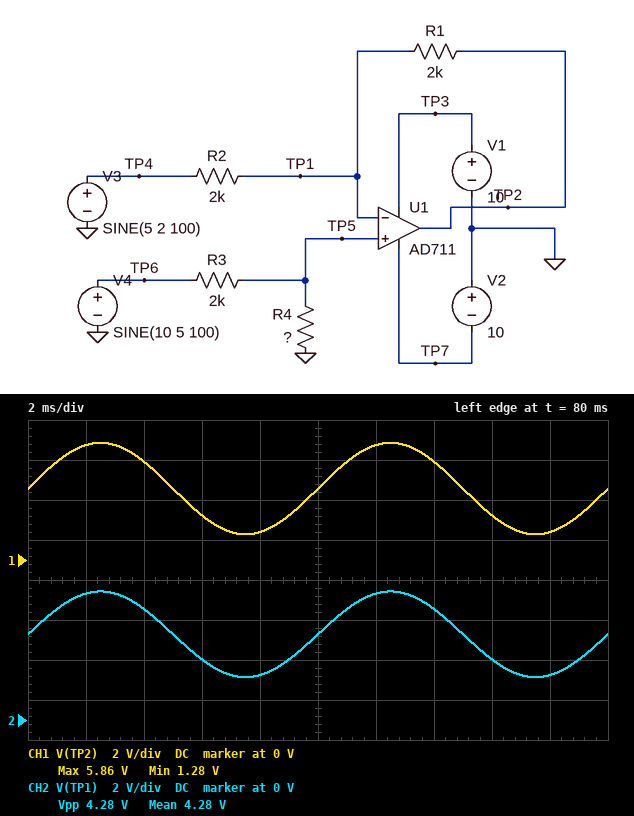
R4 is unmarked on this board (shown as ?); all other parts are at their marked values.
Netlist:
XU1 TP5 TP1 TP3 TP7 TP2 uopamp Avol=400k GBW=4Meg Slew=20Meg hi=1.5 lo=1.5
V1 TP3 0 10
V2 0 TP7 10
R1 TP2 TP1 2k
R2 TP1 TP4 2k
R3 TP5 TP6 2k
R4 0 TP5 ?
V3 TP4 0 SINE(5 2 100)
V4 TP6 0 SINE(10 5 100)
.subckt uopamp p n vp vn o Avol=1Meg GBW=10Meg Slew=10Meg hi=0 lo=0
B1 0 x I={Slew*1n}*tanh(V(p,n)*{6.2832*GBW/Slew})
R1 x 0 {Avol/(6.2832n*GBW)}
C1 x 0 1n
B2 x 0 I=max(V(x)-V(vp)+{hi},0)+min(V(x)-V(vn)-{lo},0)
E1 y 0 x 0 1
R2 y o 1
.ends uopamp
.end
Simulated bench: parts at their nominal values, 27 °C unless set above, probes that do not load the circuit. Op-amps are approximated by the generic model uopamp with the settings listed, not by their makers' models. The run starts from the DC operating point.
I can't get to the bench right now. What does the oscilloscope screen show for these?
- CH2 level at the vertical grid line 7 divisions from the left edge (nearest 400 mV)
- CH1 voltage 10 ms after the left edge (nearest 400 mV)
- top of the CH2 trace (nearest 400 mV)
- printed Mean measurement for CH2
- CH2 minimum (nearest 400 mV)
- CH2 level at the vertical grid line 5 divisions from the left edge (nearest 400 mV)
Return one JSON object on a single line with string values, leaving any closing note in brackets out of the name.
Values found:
{"CH2 level at the vertical grid line 7 divisions from the left edge": "5.6 V", "CH1 voltage 10 ms after the left edge": "3.6 V", "top of the CH2 trace": "6.4 V", "printed Mean measurement for CH2": "4.28 V", "CH2 minimum": "2.0 V", "CH2 level at the vertical grid line 5 divisions from the left edge": "4.4 V"}
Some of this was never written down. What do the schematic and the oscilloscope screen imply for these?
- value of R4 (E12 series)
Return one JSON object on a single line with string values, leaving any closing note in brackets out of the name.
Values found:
{"value of R4": "1.5 kΩ"}
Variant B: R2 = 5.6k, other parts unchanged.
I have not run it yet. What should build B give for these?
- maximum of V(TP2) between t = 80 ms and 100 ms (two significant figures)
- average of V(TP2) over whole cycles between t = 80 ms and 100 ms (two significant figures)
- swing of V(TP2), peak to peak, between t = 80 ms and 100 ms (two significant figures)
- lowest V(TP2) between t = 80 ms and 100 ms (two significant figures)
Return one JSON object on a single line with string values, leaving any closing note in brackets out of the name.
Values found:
{"maximum of V(TP2) between t = 80 ms and 100 ms": "6.2 V", "average of V(TP2) over whole cycles between t = 80 ms and 100 ms": "4.0 V", "swing of V(TP2), peak to peak, between t = 80 ms and 100 ms": "4.4 V", "lowest V(TP2) between t = 80 ms and 100 ms": "1.8 V"}
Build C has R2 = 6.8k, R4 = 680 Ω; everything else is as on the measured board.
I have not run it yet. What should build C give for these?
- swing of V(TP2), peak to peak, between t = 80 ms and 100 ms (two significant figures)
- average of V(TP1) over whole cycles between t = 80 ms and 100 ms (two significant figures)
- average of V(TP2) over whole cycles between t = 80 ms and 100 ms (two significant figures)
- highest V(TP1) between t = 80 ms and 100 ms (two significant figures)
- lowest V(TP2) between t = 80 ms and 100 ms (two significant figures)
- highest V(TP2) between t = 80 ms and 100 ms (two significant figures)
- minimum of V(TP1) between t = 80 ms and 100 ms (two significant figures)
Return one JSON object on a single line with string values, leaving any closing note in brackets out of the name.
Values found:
{"swing of V(TP2), peak to peak, between t = 80 ms and 100 ms": "2.1 V", "average of V(TP1) over whole cycles between t = 80 ms and 100 ms": "2.5 V", "average of V(TP2) over whole cycles between t = 80 ms and 100 ms": "1.8 V", "highest V(TP1) between t = 80 ms and 100 ms": "3.8 V", "lowest V(TP2) between t = 80 ms and 100 ms": "760 mV", "highest V(TP2) between t = 80 ms and 100 ms": "2.9 V", "minimum of V(TP1) between t = 80 ms and 100 ms": "1.3 V"}
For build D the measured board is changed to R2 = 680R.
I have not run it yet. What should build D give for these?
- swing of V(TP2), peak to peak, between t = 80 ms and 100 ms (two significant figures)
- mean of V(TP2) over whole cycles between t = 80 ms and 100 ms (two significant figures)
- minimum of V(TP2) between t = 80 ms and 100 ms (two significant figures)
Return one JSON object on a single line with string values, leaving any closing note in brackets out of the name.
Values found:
{"swing of V(TP2), peak to peak, between t = 80 ms and 100 ms": "5.1 V", "mean of V(TP2) over whole cycles between t = 80 ms and 100 ms": "2.2 V", "minimum of V(TP2) between t = 80 ms and 100 ms": "-380 mV"}
